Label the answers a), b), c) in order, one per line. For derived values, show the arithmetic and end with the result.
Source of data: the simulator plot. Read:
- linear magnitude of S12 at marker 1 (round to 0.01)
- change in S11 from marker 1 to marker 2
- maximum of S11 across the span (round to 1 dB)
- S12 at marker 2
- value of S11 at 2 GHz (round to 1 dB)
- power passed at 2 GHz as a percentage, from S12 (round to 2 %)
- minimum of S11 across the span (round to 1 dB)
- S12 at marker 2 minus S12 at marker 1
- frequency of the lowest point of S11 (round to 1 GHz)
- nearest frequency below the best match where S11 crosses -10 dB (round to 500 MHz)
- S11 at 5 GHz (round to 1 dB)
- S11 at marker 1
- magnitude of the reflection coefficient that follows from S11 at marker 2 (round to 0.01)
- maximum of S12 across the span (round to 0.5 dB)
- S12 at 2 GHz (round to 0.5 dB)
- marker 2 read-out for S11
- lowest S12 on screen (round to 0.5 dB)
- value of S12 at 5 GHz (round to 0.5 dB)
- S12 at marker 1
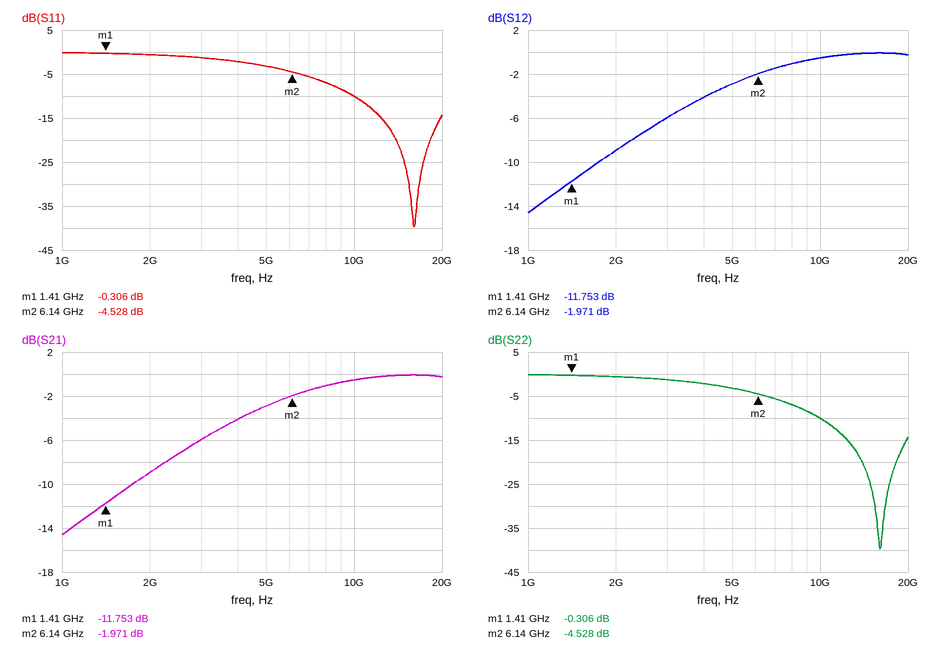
a) 10^(-11.753/20) ≈ 0.26
b) -4.528 − (-0.306) = -4.222 dB
c) 0 dB
d) -1.971 dB
e) -1 dB
f) 10^(-9/10) ≈ 12.6 %, so 12 % to the nearest 2 %
g) -40 dB
h) -1.971 − (-11.753) = 9.782 dB
i) 16 GHz
j) 10.0 GHz
k) -3 dB
l) -0.306 dB
m) 10^(-4.528/20) ≈ 0.59
n) 0.0 dB
o) -9.0 dB
p) -4.528 dB
q) -14.5 dB
r) -3.0 dB
s) -11.753 dB
